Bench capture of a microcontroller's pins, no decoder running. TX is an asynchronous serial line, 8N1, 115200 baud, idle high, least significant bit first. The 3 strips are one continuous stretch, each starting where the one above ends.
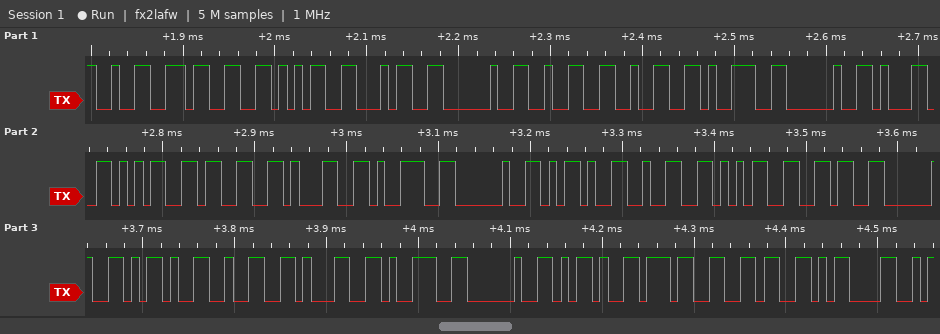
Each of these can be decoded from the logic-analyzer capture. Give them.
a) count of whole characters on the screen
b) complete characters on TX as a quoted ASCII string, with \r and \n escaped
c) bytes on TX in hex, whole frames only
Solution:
29
"2354 229 15319 -256 -219 -76\r"
32 33 35 34 20 32 32 39 20 31 35 33 31 39 20 2D 32 35 36 20 2D 32 31 39 20 2D 37 36 0D
